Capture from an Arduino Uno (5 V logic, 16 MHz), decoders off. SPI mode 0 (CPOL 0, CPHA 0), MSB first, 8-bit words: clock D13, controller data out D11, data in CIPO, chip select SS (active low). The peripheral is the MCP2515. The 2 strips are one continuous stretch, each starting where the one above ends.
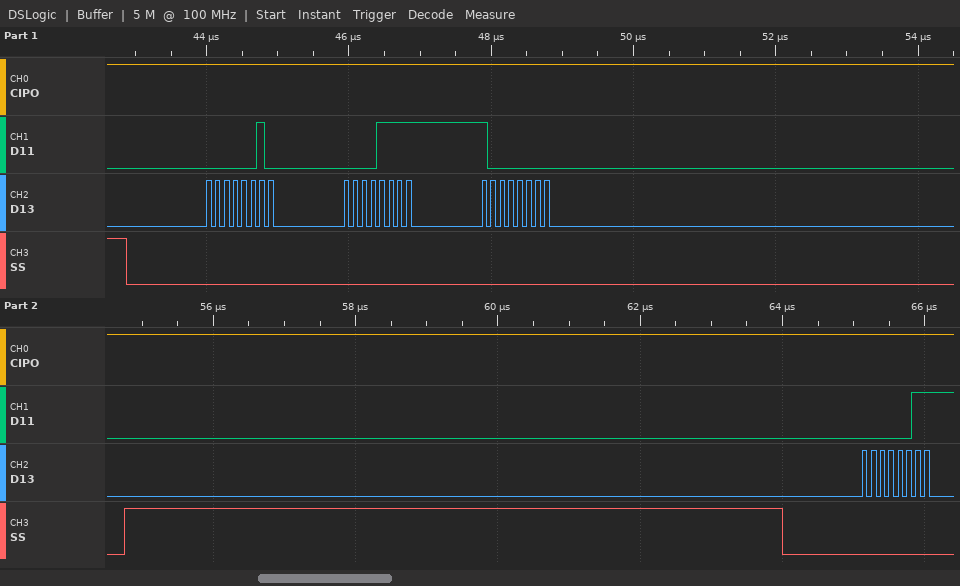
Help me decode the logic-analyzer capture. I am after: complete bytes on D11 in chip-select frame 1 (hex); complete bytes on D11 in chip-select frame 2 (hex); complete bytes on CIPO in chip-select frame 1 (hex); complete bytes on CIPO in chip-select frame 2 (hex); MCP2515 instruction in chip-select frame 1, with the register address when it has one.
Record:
02 0F 80
03
FF FF FF
FF
WRITE 0x0F
